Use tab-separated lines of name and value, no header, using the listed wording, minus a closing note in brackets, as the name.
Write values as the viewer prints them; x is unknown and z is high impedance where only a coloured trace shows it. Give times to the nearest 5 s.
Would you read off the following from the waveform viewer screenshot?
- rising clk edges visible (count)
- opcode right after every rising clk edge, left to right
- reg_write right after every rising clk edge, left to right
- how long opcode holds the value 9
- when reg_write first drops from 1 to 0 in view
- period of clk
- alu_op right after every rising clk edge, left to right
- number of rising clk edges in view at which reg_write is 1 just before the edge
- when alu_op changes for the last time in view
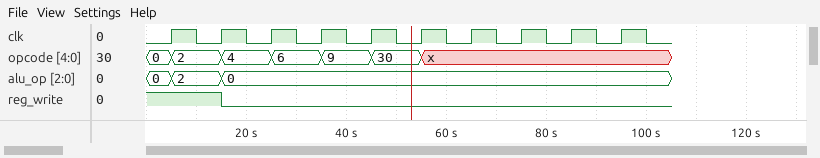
rising clk edges visible	10
opcode right after every rising clk edge, left to right	2, 4, 6, 9, 30, x, x, x, x, x
reg_write right after every rising clk edge, left to right	1 0 0 0 0 0 0 0 0 0
how long opcode holds the value 9	10 s
when reg_write first drops from 1 to 0 in view	15 s
period of clk	10 s
alu_op right after every rising clk edge, left to right	2, 0, 0, 0, 0, 0, 0, 0, 0, 0
number of rising clk edges in view at which reg_write is 1 just before the edge	2
when alu_op changes for the last time in view	15 s
